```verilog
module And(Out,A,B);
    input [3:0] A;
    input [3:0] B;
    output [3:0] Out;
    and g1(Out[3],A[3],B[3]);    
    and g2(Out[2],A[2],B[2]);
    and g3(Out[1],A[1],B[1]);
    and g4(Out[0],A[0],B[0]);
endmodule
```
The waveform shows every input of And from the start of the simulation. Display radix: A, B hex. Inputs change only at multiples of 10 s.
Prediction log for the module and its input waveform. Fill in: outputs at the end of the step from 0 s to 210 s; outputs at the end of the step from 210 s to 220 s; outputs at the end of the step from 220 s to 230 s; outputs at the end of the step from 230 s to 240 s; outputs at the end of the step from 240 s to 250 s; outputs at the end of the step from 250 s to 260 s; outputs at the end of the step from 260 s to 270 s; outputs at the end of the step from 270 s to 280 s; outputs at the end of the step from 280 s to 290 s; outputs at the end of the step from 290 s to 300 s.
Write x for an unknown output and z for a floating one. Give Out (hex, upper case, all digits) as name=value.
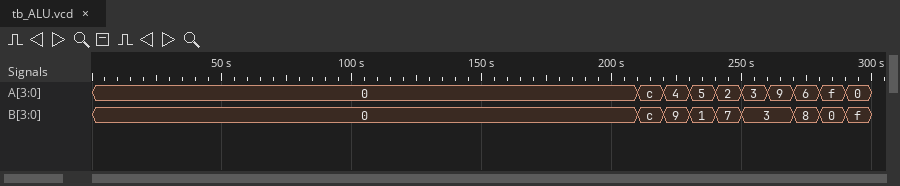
Out=0
Out=C
Out=0
Out=1
Out=2
Out=3
Out=1
Out=0
Out=0
Out=0
